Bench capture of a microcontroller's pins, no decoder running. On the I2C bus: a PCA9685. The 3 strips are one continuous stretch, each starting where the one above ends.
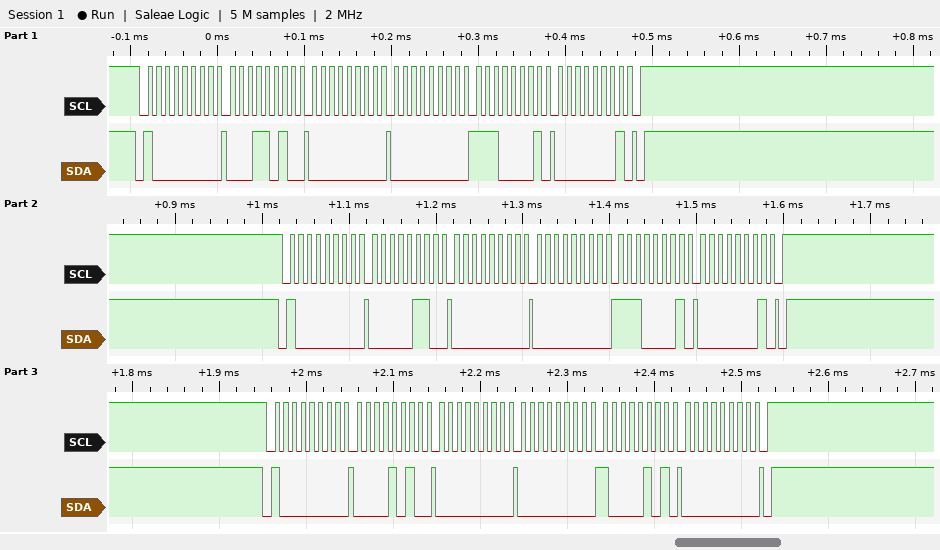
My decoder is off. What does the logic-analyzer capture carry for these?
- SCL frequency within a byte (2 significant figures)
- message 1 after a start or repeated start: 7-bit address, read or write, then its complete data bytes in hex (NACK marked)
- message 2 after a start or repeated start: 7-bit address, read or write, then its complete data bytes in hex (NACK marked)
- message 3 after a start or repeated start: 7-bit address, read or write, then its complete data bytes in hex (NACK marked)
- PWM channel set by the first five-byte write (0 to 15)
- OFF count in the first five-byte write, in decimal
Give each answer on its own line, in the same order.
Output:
100 kHz
0x40 write: 1A 00 00 E1 01
0x40 write: 06 00 00 E1 01
0x40 write: 0A 00 00 85 00
5
481
